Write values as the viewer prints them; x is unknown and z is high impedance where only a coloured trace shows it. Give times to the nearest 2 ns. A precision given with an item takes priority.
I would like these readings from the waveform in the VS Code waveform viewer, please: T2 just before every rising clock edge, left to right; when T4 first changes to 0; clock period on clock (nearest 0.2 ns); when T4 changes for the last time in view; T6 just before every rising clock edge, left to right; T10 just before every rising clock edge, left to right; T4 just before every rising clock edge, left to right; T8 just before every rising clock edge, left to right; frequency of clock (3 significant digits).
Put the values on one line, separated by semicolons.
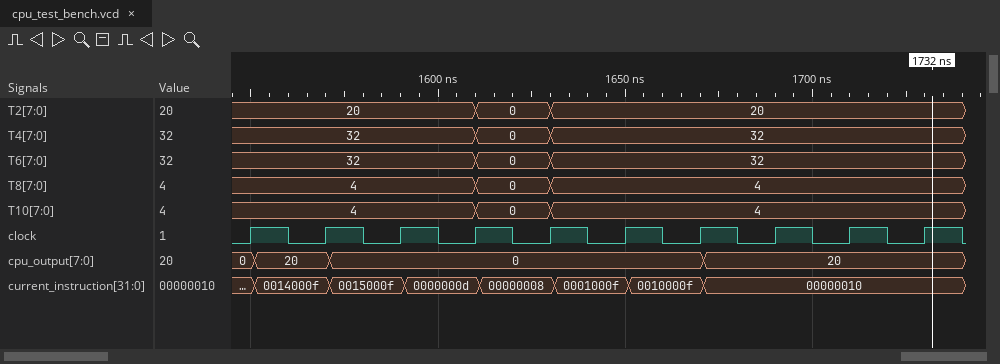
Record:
20, 20, 20, 20, 0, 20, 20, 20, 20, 20; 1610 ns; 20 ns; 1630 ns; 32, 32, 32, 32, 0, 32, 32, 32, 32, 32; 4, 4, 4, 4, 0, 4, 4, 4, 4, 4; 32, 32, 32, 32, 0, 32, 32, 32, 32, 32; 4, 4, 4, 4, 0, 4, 4, 4, 4, 4; 50.0 MHz
